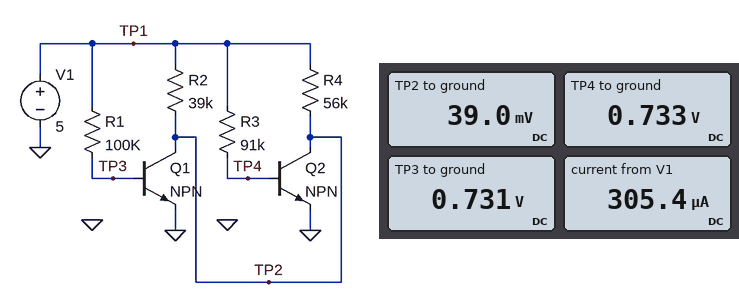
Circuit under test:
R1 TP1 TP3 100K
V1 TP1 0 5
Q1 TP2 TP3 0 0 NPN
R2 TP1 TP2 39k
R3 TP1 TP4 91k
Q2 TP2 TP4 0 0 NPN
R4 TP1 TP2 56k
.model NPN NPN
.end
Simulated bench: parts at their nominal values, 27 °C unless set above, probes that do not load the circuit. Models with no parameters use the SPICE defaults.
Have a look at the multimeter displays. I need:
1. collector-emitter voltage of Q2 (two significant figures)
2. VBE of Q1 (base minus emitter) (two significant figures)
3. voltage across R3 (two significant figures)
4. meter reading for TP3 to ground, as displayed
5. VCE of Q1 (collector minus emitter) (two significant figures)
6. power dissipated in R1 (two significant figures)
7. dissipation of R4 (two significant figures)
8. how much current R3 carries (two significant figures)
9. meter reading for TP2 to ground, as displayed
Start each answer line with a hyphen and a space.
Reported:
- 39 mV
- 730 mV
- 4.3 V
- 0.731 V
- 39 mV
- 180 µW
- 440 µW
- 47 µA
- 39.0 mV
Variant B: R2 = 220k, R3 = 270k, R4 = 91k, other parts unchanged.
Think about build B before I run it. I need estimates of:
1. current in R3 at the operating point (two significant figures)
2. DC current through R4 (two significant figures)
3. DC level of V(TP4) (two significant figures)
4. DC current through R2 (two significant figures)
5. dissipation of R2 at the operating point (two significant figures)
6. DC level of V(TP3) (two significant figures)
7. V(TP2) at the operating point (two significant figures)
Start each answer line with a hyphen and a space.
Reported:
- 16 µA
- 55 µA
- 700 mV
- 23 µA
- 110 µW
- 720 mV
- 31 mV
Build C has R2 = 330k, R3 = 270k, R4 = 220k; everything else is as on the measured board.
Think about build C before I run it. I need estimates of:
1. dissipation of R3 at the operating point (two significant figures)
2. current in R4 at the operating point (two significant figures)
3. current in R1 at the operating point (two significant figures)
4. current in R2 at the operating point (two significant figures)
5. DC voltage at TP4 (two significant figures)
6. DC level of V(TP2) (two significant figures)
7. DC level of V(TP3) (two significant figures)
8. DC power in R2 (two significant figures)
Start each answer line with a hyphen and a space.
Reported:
- 69 µW
- 23 µA
- 43 µA
- 15 µA
- 690 mV
- 25 mV
- 720 mV
- 75 µW
